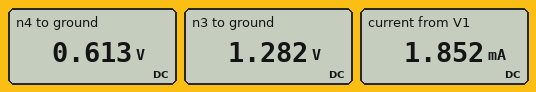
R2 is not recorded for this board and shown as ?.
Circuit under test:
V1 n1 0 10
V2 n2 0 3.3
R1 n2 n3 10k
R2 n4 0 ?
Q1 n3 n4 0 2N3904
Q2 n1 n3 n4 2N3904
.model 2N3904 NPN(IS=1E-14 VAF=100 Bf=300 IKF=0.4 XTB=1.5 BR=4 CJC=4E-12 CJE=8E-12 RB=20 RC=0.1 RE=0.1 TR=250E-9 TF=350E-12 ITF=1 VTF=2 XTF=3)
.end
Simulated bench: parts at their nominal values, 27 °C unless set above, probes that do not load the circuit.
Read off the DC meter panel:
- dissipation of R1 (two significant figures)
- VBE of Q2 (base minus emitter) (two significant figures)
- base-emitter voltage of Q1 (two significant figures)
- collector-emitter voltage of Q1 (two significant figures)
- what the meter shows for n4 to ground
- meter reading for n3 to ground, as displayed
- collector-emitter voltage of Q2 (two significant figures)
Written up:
410 µW
670 mV
610 mV
1.3 V
0.613 V
1.282 V
9.4 V
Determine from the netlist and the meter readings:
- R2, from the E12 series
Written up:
330 Ω
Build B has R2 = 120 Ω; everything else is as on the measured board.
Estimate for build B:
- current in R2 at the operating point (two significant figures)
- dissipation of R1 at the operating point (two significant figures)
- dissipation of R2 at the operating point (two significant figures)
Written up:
5.1 mA
400 µW
3.1 mW
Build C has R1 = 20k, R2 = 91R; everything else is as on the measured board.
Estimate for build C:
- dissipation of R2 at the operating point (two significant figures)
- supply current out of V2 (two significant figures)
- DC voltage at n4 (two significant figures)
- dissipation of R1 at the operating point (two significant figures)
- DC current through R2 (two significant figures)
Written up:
3.8 mW
100 µA
590 mV
200 µW
6.5 mA
